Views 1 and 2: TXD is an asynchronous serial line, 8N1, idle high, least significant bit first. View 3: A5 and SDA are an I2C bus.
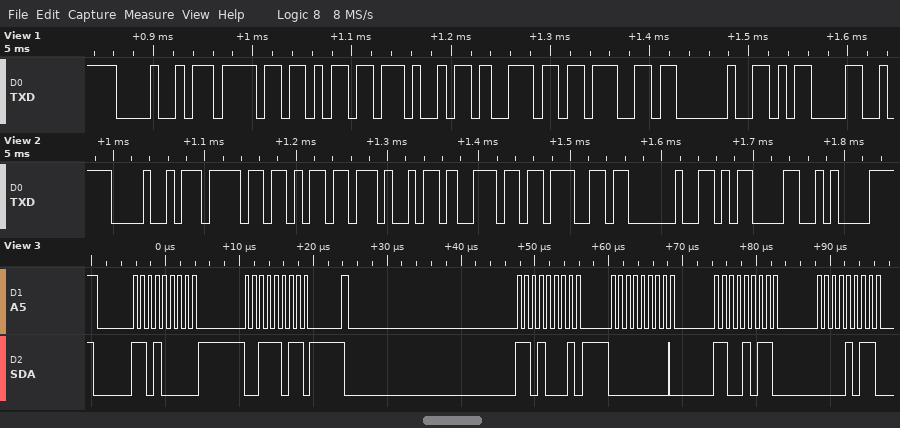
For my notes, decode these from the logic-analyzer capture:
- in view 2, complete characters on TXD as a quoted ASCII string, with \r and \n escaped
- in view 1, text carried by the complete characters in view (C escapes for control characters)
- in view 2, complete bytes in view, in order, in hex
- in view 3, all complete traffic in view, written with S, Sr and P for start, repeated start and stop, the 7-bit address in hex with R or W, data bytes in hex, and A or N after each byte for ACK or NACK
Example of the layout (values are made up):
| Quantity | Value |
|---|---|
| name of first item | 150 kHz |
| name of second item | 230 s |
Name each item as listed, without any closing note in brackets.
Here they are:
| Quantity | Value |
|---|---|
| in view 2, complete characters on TXD as a quoted ASCII string, with \r and \n escaped | "Homing \r\n" |
| in view 1, text carried by the complete characters in view | "Homing \r" |
| in view 2, complete bytes in view, in order, in hex | 0x48 0x6F 0x6D 0x69 0x6E 0x67 0x20 0x0D 0x0A |
| in view 3, all complete traffic in view, written with S, Sr and P for start, repeated start and stop, the 7-bit address in hex with R or W, data bytes in hex, and A or N after each byte for ACK or NACK | S 68W A 3B A Sr 68R A 00 A CB A 0B A |
